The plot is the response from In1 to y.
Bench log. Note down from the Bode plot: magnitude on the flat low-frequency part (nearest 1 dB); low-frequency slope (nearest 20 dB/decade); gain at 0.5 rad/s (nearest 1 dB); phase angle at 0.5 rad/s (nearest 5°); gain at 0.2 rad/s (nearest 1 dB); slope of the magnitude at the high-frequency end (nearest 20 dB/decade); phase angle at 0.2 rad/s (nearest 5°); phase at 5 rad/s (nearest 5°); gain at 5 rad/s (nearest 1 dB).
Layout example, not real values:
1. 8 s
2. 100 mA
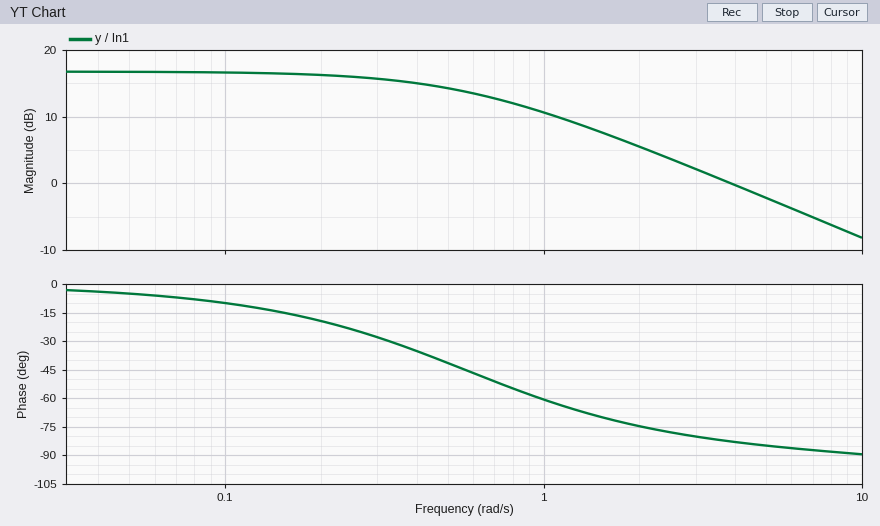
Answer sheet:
1. 17 dB
2. 0 dB/decade
3. 14 dB
4. -40°
5. 16 dB
6. -20 dB/decade
7. -20°
8. -85°
9. -2 dB
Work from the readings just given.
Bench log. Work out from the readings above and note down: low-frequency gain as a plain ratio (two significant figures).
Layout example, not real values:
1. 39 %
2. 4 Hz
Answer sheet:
1. 7.1
